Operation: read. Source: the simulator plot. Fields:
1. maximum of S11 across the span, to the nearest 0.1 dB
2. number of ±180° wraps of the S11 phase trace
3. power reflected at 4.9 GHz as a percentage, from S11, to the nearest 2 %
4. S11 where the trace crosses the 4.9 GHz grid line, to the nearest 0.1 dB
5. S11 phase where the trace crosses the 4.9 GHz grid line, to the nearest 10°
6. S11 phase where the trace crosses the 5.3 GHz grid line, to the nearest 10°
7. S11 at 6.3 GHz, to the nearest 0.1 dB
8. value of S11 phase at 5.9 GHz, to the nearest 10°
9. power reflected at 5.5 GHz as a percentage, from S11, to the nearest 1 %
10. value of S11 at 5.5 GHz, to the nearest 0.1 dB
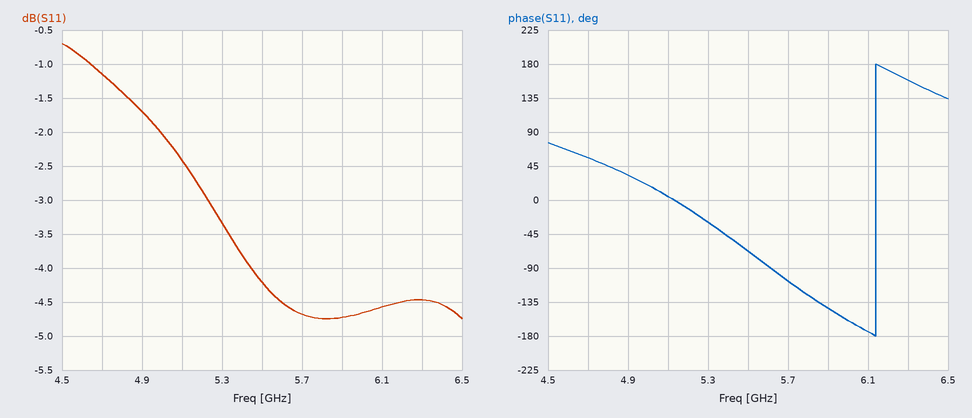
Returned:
-0.7 dB
1
68 %
-1.7 dB
30°
-30°
-4.5 dB
-140°
38 %
-4.2 dB
